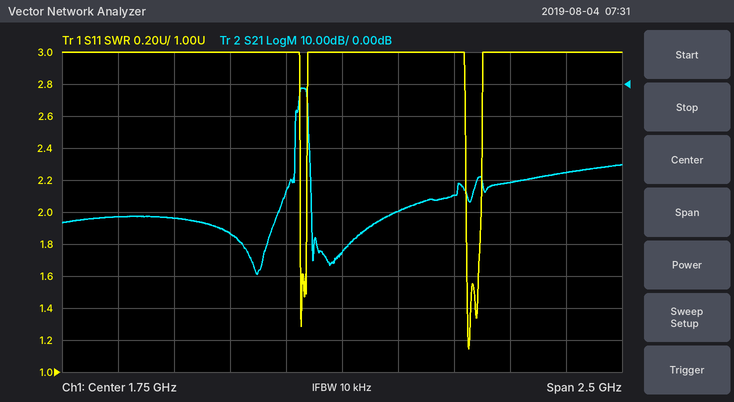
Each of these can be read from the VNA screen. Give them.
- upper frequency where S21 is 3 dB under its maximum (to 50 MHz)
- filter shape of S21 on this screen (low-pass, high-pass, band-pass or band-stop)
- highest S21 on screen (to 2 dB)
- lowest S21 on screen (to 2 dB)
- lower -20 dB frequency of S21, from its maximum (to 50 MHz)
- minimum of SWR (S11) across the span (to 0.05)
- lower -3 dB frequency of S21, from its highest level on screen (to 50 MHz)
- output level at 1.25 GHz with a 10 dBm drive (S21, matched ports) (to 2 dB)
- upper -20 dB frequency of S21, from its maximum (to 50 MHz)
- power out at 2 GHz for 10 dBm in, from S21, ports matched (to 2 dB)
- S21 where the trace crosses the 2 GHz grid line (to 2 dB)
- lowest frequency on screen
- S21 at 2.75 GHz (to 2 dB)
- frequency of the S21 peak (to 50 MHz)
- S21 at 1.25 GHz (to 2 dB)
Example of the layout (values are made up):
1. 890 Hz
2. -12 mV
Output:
1. 1.60 GHz
2. band-pass
3. -2 dB
4. -60 dB
5. 1.55 GHz
6. 1.15
7. 1.55 GHz
8. -36 dBm
9. 1.60 GHz
10. -30 dBm
11. -40 dB
12. 500 MHz
13. -28 dB
14. 1.55 GHz
15. -46 dB
